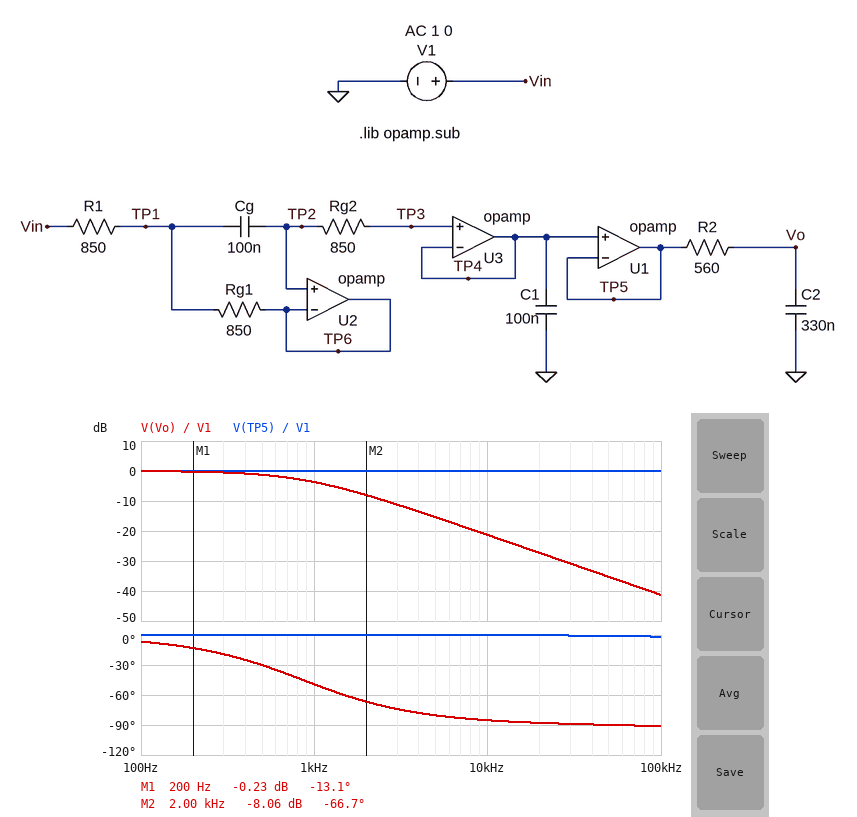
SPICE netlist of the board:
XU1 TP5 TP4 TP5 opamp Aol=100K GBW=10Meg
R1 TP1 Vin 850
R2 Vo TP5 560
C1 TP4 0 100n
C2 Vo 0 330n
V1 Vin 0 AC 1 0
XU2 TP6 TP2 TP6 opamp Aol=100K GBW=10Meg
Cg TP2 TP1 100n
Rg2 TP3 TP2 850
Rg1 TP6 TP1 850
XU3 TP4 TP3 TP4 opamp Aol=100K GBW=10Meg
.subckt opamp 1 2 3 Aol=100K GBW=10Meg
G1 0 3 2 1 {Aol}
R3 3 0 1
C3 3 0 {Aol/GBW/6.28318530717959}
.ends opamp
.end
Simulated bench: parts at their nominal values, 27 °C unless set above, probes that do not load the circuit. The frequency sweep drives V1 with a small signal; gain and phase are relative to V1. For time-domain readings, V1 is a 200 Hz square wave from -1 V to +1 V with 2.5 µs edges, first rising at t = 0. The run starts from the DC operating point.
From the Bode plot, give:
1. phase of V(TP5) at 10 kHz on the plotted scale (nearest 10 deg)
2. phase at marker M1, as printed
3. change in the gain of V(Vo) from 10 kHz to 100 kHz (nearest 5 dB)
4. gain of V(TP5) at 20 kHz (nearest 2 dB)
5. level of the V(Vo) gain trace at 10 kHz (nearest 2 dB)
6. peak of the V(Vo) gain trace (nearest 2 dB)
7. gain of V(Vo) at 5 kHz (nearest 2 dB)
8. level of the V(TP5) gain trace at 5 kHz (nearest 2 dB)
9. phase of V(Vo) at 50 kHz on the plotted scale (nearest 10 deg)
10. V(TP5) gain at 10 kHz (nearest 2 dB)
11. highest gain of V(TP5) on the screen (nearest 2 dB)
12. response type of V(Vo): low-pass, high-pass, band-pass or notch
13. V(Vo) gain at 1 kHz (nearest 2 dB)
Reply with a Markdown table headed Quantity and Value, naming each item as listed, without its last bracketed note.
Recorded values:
| Quantity | Value |
|---|---|
| phase of V(TP5) at 10 kHz on the plotted scale | 0 deg |
| phase at marker M1, as printed | -13.1 deg |
| change in the gain of V(Vo) from 10 kHz to 100 kHz | -20 dB |
| gain of V(TP5) at 20 kHz | 0 dB |
| level of the V(Vo) gain trace at 10 kHz | -22 dB |
| peak of the V(Vo) gain trace | 0 dB |
| gain of V(Vo) at 5 kHz | -16 dB |
| level of the V(TP5) gain trace at 5 kHz | 0 dB |
| phase of V(Vo) at 50 kHz on the plotted scale | -90 deg |
| V(TP5) gain at 10 kHz | 0 dB |
| highest gain of V(TP5) on the screen | 0 dB |
| response type of V(Vo): low-pass, high-pass, band-pass or notch | low-pass |
| V(Vo) gain at 1 kHz | -4 dB |
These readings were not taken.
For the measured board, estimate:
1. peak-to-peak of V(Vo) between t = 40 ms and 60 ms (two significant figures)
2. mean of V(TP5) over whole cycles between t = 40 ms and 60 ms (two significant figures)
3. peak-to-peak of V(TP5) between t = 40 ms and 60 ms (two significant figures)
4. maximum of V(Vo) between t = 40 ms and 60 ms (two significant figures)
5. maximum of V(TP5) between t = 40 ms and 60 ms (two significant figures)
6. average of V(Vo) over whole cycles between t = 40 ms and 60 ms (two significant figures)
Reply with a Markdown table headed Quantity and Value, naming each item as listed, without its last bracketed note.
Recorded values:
| Quantity | Value |
|---|---|
| peak-to-peak of V(Vo) between t = 40 ms and 60 ms | 2.0 V |
| mean of V(TP5) over whole cycles between t = 40 ms and 60 ms | 1.0 V |
| peak-to-peak of V(TP5) between t = 40 ms and 60 ms | 2.0 V |
| maximum of V(Vo) between t = 40 ms and 60 ms | 2.0 V |
| maximum of V(TP5) between t = 40 ms and 60 ms | 2.0 V |
| average of V(Vo) over whole cycles between t = 40 ms and 60 ms | 1.0 V |
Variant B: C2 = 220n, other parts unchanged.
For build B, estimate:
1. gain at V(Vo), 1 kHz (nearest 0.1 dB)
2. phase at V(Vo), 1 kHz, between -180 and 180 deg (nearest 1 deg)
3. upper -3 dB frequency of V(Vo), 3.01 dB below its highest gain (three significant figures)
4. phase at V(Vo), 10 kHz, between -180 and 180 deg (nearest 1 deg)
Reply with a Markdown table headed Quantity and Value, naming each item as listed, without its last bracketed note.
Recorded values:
| Quantity | Value |
|---|---|
| gain at V(Vo), 1 kHz | -2.0 dB |
| phase at V(Vo), 1 kHz, between -180 and 180 deg | -38 deg |
| upper -3 dB frequency of V(Vo), 3.01 dB below its highest gain | 1.29 kHz |
| phase at V(Vo), 10 kHz, between -180 and 180 deg | -83 deg |
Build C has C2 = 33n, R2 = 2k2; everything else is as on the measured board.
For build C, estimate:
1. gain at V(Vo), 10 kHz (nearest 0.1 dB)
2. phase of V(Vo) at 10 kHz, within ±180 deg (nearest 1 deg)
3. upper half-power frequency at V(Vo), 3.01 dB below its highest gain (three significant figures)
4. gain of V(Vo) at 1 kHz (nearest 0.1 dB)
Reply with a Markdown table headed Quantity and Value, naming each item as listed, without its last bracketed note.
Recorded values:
| Quantity | Value |
|---|---|
| gain at V(Vo), 10 kHz | -13.4 dB |
| phase of V(Vo) at 10 kHz, within ±180 deg | -78 deg |
| upper half-power frequency at V(Vo), 3.01 dB below its highest gain | 2.19 kHz |
| gain of V(Vo) at 1 kHz | -0.8 dB |
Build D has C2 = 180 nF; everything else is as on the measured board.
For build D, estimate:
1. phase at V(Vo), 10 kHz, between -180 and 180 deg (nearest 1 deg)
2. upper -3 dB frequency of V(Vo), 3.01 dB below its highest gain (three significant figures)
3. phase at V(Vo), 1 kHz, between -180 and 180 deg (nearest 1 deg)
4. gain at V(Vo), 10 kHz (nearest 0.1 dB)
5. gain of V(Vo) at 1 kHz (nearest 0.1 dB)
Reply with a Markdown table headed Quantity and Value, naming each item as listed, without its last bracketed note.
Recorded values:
| Quantity | Value |
|---|---|
| phase at V(Vo), 10 kHz, between -180 and 180 deg | -81 deg |
| upper -3 dB frequency of V(Vo), 3.01 dB below its highest gain | 1.58 kHz |
| phase at V(Vo), 1 kHz, between -180 and 180 deg | -32 deg |
| gain at V(Vo), 10 kHz | -16.1 dB |
| gain of V(Vo) at 1 kHz | -1.5 dB |
